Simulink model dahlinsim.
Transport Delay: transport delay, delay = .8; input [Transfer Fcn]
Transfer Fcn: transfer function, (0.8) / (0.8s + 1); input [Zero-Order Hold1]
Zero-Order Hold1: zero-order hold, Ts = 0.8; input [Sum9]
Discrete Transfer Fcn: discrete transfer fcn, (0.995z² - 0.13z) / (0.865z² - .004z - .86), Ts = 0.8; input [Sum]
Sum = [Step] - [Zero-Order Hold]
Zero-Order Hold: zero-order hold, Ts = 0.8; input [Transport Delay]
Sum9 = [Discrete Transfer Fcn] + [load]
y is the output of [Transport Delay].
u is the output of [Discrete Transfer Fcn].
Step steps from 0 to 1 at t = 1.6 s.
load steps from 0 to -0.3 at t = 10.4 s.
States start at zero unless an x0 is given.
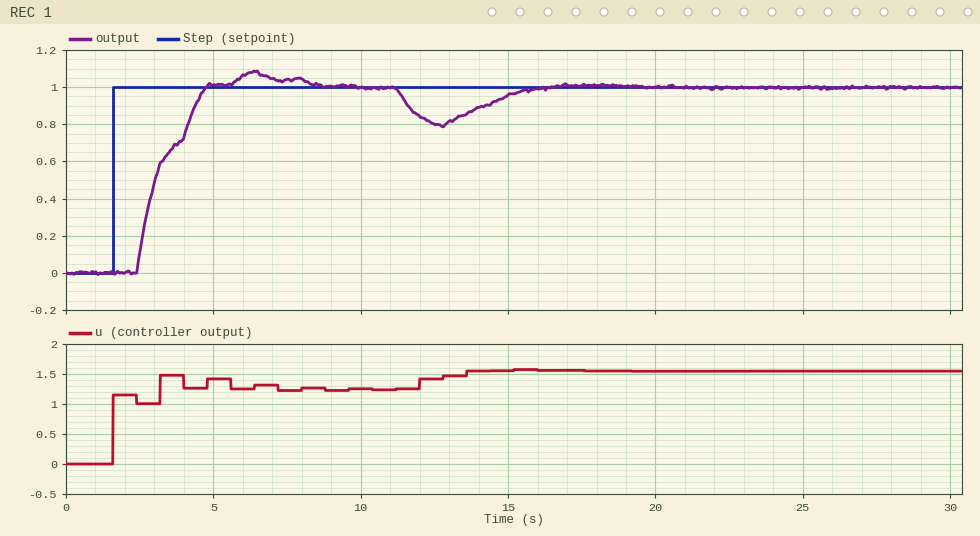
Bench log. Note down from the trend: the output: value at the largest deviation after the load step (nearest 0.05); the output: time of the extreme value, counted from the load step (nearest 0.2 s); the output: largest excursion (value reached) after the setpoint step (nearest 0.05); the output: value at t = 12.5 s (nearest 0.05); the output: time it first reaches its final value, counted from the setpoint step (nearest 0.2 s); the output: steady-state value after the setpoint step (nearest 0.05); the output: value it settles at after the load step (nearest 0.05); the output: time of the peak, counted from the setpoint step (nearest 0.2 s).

0.80
2.4 s
1.10
0.80
3.2 s
1.00
1.00
4.8 s
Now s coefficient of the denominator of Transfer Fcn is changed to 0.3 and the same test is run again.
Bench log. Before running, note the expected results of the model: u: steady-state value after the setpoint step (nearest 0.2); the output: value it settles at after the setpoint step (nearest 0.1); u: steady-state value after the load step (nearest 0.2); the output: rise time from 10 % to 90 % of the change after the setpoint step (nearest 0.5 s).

1.2
1.0
1.6
2.0 s
